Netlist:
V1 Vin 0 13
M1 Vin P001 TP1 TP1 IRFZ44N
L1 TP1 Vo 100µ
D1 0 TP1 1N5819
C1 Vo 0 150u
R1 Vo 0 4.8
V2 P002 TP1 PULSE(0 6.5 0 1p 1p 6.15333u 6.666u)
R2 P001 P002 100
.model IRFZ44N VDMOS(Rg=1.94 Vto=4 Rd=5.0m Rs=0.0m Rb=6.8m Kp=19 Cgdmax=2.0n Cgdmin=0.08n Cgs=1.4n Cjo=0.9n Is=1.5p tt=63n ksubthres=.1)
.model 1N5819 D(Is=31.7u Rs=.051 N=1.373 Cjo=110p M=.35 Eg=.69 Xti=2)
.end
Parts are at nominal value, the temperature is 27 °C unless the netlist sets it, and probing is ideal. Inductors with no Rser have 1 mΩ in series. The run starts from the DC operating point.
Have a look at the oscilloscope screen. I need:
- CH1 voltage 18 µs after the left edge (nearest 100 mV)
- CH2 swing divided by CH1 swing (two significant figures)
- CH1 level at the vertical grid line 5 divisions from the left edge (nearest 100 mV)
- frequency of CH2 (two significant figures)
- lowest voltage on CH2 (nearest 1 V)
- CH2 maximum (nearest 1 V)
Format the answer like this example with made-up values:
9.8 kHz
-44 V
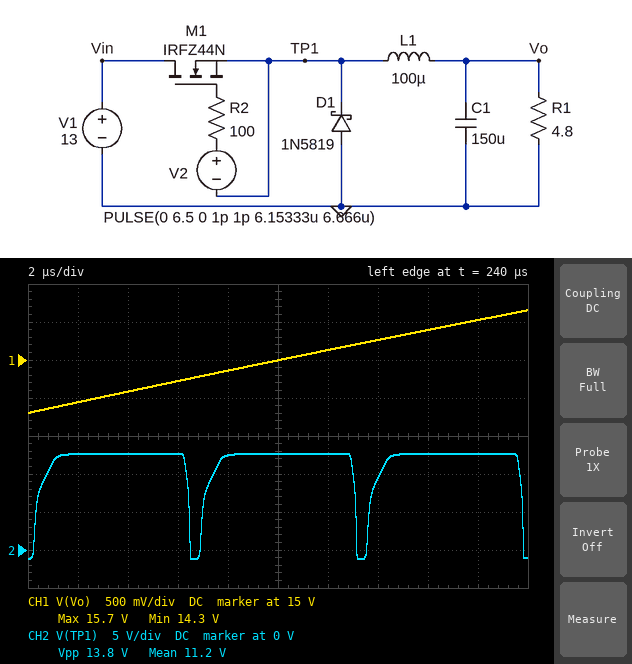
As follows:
15.5 V
10
15.0 V
150 kHz
-1 V
13 V
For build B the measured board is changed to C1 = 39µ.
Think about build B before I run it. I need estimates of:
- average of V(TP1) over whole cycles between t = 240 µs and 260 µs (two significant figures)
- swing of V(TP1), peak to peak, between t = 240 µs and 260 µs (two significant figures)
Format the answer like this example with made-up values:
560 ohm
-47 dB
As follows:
12 V
13 V
